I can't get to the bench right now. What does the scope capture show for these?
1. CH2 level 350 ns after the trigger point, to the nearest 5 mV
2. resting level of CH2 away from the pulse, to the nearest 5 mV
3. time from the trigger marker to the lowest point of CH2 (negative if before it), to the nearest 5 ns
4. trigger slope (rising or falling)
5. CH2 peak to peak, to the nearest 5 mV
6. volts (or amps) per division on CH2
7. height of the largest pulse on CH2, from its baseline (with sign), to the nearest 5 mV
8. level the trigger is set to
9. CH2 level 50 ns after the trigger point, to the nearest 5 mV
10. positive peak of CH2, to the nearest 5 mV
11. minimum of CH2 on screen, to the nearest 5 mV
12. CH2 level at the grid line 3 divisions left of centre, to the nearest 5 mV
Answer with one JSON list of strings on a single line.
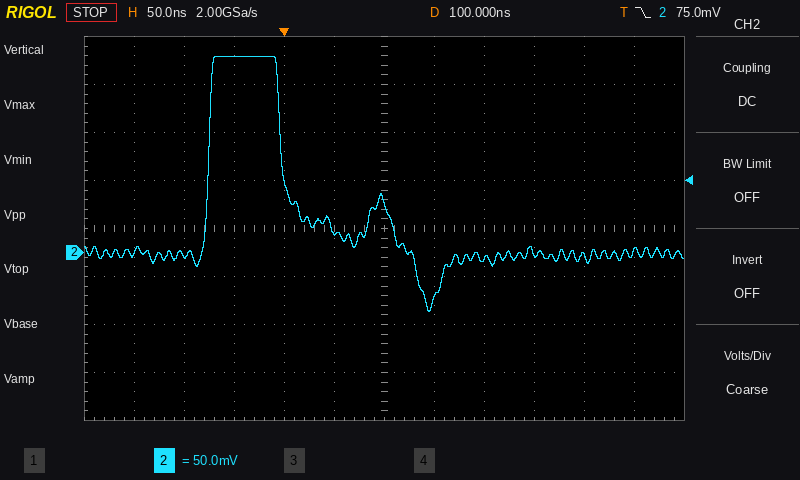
["0 mV", "0 mV", "+145 ns", "falling", "265 mV", "50 mV", "+205 mV", "75.0 mV", "20 mV", "205 mV", "-60 mV", "205 mV"]
